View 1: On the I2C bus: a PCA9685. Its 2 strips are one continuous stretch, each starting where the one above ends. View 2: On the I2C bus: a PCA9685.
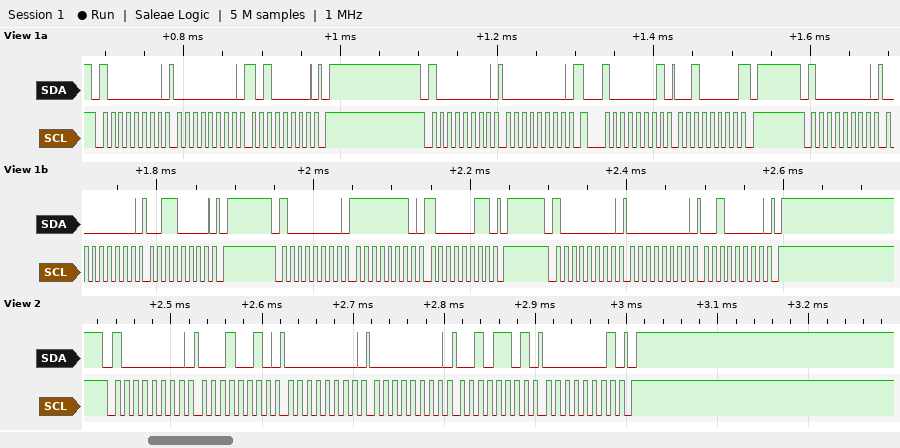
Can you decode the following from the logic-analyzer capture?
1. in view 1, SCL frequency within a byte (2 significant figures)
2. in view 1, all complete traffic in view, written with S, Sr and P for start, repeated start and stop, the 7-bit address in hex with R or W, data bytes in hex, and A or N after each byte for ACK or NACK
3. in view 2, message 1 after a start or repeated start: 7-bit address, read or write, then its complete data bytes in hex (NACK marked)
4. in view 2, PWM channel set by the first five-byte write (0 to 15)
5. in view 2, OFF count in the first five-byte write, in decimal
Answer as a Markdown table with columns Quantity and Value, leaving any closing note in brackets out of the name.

| Quantity | Value |
|---|---|
| in view 1, SCL frequency within a byte | 100 kHz |
| in view 1, all complete traffic in view, written with S, Sr and P for start, repeated start and stop, the 7-bit address in hex with R or W, data bytes in hex, and A or N after each byte for ACK or NACK | S 40W A 00 A A0 A P S 40W A 00 A Sr 40R A 20 N P S 40W A 00 A 30 A P S 40W A FE A 83 A P S 40W A 00 A 20 A P |
| in view 2, message 1 after a start or repeated start: 7-bit address, read or write, then its complete data bytes in hex | 0x40 write: 12 00 00 2D 01 |
| in view 2, PWM channel set by the first five-byte write | 3 |
| in view 2, OFF count in the first five-byte write, in decimal | 301 |
